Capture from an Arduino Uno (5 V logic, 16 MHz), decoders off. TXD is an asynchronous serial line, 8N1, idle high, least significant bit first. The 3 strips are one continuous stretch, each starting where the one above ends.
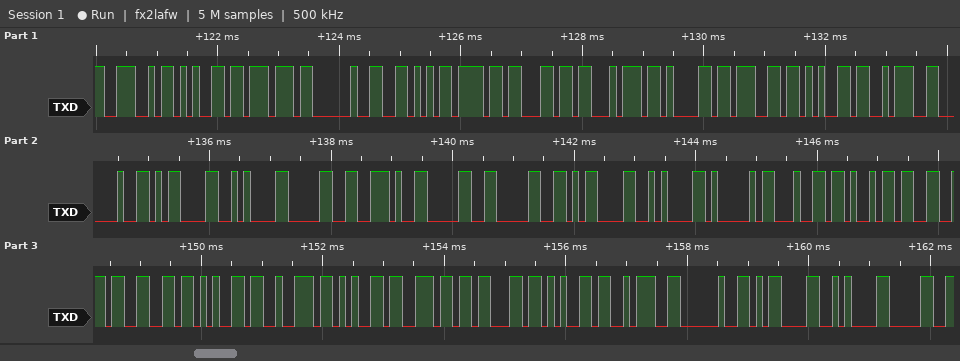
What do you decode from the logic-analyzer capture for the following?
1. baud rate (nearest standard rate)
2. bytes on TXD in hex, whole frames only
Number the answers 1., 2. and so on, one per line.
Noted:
1. 9600 baud
2. 4E 65 77 20 56 6F 6C 74 61 67 65 3A 20 0D 0A 30 2E 30 30 0D 0A 41 64 69 66 66 65 72 65 6E 63 65 3A 20 0D 0A 30
